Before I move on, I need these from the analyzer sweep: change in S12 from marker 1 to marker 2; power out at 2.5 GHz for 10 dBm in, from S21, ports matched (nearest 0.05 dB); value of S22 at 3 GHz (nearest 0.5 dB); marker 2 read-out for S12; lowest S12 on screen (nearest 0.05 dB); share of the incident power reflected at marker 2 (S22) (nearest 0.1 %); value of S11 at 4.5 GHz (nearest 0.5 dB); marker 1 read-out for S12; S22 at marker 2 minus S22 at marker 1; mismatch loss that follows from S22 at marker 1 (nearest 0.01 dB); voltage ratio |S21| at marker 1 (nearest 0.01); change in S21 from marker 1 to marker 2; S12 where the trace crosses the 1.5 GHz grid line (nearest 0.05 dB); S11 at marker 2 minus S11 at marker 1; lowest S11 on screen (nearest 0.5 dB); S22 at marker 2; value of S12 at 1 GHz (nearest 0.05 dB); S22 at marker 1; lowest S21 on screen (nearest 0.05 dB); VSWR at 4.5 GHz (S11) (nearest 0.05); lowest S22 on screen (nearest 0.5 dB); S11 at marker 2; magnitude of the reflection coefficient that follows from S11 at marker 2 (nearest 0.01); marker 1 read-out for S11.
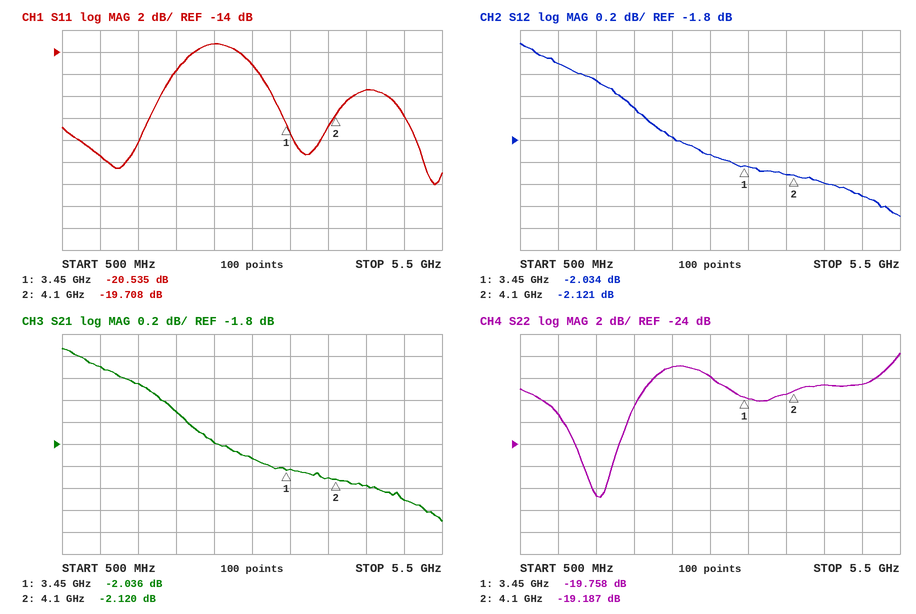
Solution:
-0.087 dB
8.20 dBm
-18.0 dB
-2.121 dB
-2.50 dB
1.2 %
-17.5 dB
-2.034 dB
0.571 dB
0.05 dB
0.79
-0.084 dB
-1.25 dB
0.827 dB
-26.0 dB
-19.187 dB
-1.10 dB
-19.758 dB
-2.50 dB
1.30
-29.0 dB
-19.708 dB
0.10
-20.535 dB
